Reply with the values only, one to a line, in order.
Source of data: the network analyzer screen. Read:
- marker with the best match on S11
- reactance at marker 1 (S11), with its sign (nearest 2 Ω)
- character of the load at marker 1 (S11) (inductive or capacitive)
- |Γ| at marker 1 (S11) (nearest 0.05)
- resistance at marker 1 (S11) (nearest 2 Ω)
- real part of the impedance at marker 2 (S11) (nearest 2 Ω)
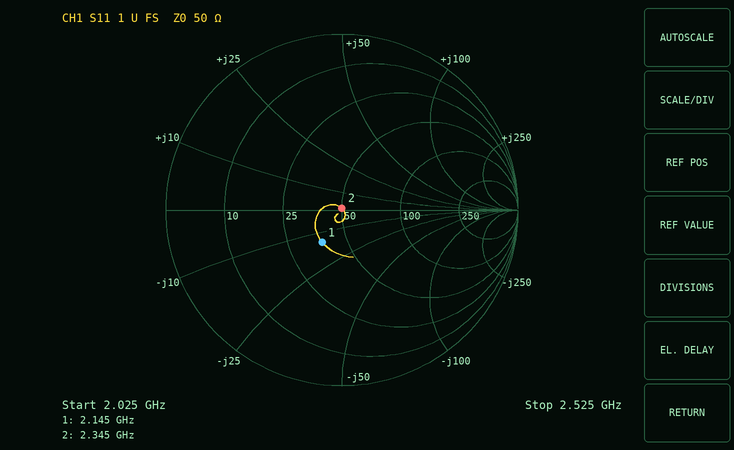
marker 2
-14 Ω
capacitive
0.20
38 Ω
50 Ω
